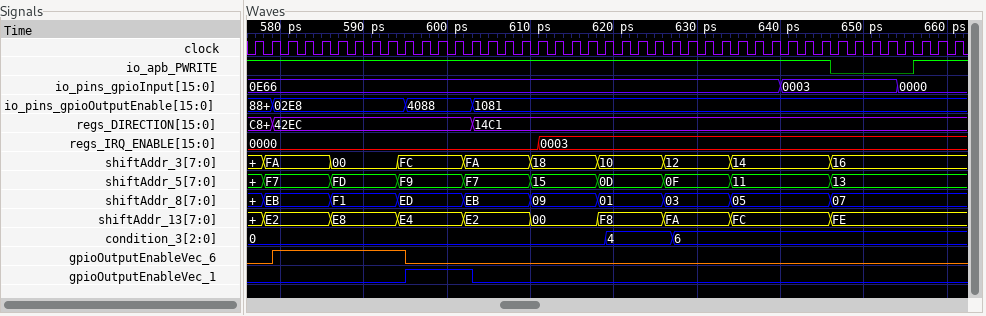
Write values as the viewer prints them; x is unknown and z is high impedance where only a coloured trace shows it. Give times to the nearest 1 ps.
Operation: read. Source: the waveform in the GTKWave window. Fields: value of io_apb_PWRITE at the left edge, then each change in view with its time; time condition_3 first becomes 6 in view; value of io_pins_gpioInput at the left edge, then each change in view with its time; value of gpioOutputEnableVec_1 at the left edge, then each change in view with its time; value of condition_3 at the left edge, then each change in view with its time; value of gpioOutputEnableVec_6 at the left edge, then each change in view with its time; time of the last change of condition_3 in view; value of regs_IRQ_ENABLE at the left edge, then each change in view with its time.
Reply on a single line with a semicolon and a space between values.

1, 0 at 646 ps, 1 at 656 ps; 627 ps; 0E66, 0003 at 640 ps, 0000 at 654 ps; 0, 1 at 595 ps, 0 at 603 ps; 0, 4 at 619 ps, 6 at 627 ps; 0, 1 at 579 ps, 0 at 595 ps; 627 ps; 0000, 0003 at 611 ps
